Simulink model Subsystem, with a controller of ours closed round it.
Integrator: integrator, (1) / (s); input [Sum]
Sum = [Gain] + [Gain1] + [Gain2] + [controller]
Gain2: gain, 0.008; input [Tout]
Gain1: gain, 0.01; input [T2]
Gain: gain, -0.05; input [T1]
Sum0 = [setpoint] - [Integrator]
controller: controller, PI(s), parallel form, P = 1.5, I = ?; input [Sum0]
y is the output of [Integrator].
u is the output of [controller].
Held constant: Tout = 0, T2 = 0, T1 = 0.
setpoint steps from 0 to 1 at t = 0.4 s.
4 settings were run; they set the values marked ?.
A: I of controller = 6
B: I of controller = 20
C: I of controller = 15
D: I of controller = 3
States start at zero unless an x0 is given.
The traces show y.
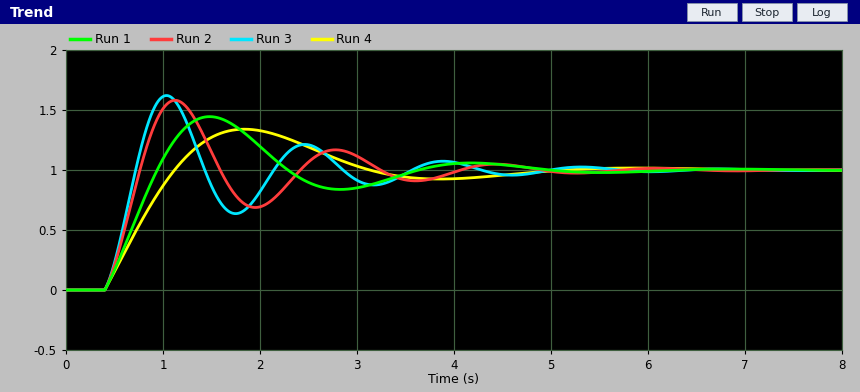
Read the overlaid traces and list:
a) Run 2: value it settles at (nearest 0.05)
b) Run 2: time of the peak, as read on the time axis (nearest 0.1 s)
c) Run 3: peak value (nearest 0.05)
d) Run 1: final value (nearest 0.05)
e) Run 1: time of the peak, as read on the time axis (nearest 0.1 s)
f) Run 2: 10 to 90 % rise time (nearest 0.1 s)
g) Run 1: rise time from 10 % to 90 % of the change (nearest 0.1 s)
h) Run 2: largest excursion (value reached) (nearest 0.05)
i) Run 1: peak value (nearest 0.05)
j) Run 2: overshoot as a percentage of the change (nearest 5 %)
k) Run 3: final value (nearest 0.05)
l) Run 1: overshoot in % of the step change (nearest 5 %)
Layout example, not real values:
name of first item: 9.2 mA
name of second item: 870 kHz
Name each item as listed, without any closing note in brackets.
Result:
Run 2: value it settles at: 1.00
Run 2: time of the peak, as read on the time axis: 1.1 s
Run 3: peak value: 1.60
Run 1: final value: 1.00
Run 1: time of the peak, as read on the time axis: 1.5 s
Run 2: 10 to 90 % rise time: 0.3 s
Run 1: rise time from 10 % to 90 % of the change: 0.4 s
Run 2: largest excursion (value reached): 1.60
Run 1: peak value: 1.45
Run 2: overshoot as a percentage of the change: 60 %
Run 3: final value: 1.00
Run 1: overshoot in % of the step change: 45 %
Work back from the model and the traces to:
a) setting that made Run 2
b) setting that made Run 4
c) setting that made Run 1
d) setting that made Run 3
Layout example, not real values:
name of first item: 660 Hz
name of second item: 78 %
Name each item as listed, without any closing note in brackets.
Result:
setting that made Run 2: C
setting that made Run 4: D
setting that made Run 1: A
setting that made Run 3: B
